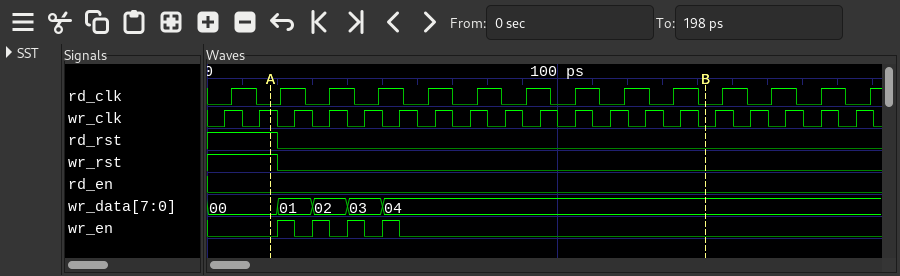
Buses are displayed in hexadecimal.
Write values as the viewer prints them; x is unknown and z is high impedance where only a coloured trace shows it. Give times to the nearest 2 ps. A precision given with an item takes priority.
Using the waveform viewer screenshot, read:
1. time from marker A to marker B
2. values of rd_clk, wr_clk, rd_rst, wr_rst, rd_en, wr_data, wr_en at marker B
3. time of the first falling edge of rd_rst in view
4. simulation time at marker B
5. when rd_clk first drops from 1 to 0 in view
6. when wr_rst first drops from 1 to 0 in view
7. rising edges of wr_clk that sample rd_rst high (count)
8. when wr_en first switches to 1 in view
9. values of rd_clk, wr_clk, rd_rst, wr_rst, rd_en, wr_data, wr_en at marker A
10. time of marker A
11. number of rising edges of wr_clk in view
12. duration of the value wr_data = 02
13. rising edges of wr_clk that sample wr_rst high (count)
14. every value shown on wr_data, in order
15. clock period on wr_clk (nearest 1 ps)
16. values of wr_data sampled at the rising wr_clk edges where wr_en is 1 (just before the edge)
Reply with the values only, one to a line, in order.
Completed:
124 ps
rd_clk=0, wr_clk=0, rd_rst=0, wr_rst=0, rd_en=0, wr_data=04, wr_en=0
20 ps
142 ps
14 ps
20 ps
2
20 ps
rd_clk=0, wr_clk=1, rd_rst=1, wr_rst=1, rd_en=0, wr_data=00, wr_en=0
18 ps
19
10 ps
2
00, 01, 02, 03, 04
10 ps
01, 02, 03, 04
